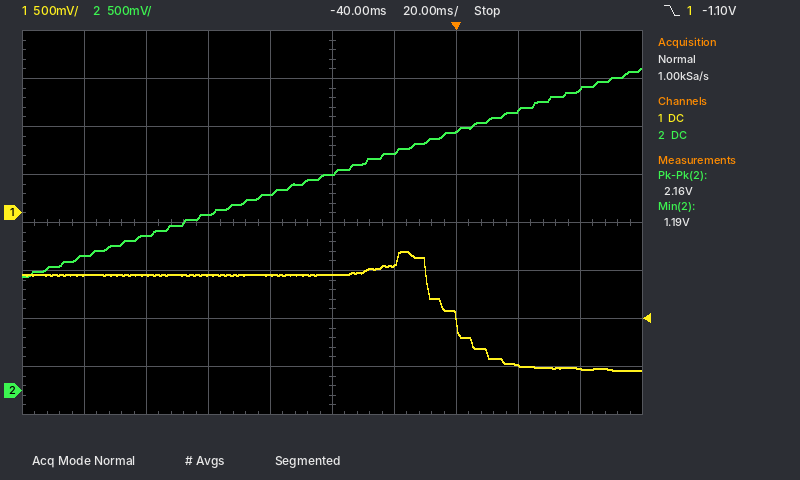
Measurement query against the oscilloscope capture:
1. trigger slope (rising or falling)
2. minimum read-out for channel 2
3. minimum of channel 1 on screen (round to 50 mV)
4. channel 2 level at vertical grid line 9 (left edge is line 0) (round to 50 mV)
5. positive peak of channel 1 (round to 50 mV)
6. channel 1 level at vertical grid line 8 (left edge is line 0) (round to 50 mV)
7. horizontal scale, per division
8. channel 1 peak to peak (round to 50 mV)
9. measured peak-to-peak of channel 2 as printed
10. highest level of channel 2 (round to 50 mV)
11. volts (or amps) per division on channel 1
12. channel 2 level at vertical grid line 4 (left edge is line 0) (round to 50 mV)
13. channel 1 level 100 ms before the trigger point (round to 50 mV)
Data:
falling
1.19 V
-1.65 V
3.15 V
-400 mV
-1.60 V
20 ms
1.25 V
2.16 V
3.35 V
500 mV
2.05 V
-650 mV
